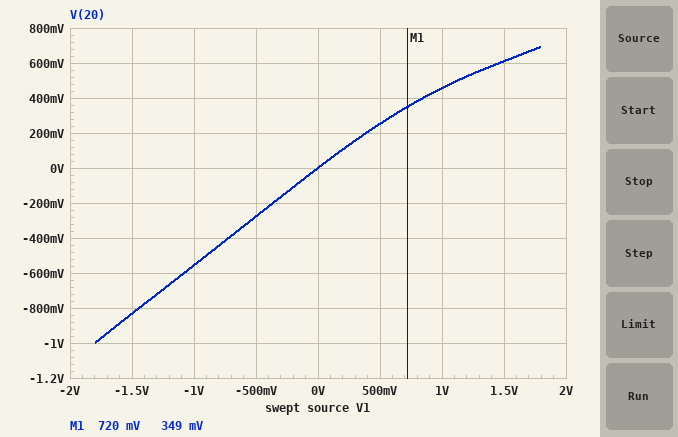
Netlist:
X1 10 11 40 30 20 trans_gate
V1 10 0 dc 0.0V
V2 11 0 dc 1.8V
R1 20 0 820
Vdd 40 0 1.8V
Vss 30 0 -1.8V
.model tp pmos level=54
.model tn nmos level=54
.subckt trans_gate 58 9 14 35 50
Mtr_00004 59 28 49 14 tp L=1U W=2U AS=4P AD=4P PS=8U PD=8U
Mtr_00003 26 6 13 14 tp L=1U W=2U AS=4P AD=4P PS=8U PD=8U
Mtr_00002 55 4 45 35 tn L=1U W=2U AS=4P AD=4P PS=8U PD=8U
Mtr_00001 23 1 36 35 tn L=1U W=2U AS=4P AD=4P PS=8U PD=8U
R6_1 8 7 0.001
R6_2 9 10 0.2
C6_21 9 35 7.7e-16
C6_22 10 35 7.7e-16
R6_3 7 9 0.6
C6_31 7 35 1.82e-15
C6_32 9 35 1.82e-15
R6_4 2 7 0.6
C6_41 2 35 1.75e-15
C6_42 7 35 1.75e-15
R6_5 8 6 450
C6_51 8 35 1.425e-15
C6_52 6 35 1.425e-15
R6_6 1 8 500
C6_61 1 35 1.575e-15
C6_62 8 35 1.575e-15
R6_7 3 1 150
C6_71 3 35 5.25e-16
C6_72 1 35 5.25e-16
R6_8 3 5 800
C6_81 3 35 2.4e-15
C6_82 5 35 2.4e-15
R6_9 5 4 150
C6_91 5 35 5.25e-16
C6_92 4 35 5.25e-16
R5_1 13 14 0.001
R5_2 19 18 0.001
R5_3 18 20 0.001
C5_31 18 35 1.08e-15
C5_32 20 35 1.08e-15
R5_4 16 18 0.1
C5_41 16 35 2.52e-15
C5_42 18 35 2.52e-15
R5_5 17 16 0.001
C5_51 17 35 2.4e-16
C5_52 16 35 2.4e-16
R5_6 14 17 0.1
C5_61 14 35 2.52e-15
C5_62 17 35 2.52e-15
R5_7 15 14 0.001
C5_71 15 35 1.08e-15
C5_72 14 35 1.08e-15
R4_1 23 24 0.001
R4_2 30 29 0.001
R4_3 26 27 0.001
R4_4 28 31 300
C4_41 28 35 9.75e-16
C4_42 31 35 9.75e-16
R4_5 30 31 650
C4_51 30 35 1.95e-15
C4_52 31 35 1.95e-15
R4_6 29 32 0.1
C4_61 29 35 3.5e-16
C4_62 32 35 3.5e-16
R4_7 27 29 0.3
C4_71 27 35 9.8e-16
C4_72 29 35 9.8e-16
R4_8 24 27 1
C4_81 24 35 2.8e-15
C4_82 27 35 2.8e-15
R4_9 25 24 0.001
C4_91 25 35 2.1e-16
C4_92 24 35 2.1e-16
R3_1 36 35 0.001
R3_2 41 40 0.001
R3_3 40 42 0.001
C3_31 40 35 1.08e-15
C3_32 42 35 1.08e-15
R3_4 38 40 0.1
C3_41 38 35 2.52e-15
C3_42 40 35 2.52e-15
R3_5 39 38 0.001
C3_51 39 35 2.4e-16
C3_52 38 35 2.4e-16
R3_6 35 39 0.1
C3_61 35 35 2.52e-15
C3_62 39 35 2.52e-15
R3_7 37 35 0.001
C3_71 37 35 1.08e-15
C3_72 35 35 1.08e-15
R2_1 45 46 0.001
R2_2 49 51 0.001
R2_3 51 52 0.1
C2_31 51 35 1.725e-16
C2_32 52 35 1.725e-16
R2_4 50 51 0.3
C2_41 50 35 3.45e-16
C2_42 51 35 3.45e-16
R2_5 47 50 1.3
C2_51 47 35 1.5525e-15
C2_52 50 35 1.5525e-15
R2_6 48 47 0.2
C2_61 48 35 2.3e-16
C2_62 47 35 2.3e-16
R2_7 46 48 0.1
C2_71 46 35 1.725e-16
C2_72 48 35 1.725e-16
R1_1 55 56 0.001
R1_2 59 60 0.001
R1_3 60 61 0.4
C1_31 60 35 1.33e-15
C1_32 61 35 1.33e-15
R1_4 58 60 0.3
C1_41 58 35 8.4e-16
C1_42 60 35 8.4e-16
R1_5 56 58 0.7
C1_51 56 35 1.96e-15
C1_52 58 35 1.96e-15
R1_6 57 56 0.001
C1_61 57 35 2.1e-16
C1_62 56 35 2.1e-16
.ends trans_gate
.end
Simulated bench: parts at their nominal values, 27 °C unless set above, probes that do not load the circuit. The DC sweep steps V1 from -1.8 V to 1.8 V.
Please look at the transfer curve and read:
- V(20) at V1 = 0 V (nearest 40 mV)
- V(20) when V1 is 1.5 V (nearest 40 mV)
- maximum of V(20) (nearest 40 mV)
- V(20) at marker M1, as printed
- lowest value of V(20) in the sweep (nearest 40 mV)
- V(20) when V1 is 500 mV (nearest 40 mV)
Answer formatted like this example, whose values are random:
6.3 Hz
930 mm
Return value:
0 V
600 mV
680 mV
349 mV
-1.00 V
240 mV
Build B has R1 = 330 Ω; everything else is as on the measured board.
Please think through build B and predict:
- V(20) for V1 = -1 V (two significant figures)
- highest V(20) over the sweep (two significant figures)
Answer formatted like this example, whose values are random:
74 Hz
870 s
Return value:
-320 mV
380 mV
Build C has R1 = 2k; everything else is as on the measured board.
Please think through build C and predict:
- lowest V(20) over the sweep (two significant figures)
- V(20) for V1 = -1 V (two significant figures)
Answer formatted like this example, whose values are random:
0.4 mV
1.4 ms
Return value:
-1.4 V
-760 mV
